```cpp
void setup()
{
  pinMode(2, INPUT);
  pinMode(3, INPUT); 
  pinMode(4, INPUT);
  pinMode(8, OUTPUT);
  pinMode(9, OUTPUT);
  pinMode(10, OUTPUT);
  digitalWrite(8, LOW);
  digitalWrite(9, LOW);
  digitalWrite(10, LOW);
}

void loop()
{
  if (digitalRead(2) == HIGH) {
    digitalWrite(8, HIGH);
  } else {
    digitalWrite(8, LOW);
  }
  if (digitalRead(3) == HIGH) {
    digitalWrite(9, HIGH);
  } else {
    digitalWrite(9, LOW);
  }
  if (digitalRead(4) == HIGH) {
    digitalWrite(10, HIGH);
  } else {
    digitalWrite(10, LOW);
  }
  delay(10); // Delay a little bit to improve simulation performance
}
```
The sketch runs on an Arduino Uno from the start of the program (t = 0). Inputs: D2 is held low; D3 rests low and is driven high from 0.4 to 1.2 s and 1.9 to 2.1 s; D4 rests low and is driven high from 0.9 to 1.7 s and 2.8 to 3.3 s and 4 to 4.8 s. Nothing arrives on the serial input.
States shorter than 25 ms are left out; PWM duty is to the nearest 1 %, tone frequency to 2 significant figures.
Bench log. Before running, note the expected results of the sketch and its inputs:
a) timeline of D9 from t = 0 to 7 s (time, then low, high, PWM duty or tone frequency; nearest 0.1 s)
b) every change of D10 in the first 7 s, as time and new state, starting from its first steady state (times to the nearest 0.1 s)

0 s low; 0.4 s high; 1.2 s low; 1.9 s high; 2.1 s low
0 s low; 0.9 s high; 1.7 s low; 2.8 s high; 3.3 s low; 4 s high; 4.8 s low
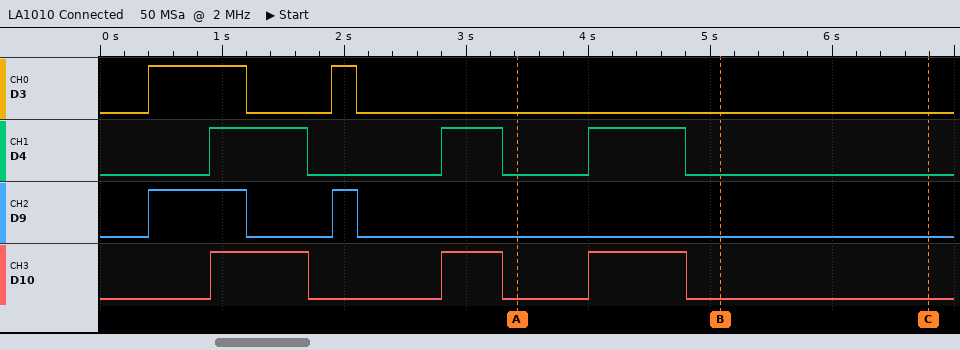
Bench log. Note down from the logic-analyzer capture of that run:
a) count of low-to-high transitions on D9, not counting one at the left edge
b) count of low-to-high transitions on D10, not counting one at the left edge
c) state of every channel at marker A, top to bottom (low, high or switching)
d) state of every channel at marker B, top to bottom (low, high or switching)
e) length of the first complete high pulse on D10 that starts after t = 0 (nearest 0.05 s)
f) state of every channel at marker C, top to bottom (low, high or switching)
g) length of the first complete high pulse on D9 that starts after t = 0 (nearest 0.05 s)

2
3
D3 low, D4 low, D9 low, D10 low
D3 low, D4 low, D9 low, D10 low
0.80 s
D3 low, D4 low, D9 low, D10 low
0.80 s
